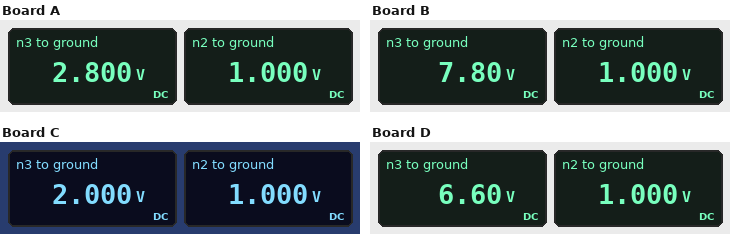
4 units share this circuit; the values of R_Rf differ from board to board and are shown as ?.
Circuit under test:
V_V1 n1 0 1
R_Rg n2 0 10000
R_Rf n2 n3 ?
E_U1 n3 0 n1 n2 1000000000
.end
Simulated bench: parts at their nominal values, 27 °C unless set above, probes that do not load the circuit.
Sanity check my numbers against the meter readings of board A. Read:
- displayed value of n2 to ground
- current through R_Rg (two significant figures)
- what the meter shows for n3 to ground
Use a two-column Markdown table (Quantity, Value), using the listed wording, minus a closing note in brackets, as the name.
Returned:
| Quantity | Value |
|---|---|
| displayed value of n2 to ground | 1.000 V |
| current through R_Rg | 100 µA |
| what the meter shows for n3 to ground | 2.800 V |
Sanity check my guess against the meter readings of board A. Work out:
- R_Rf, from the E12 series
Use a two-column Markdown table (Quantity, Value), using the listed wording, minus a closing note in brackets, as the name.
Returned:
| Quantity | Value |
|---|---|
| R_Rf, from the E12 series | 18 kΩ |
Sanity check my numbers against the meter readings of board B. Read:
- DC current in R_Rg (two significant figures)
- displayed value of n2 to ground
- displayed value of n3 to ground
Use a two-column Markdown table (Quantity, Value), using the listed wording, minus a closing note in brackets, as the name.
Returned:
| Quantity | Value |
|---|---|
| DC current in R_Rg | 100 µA |
| displayed value of n2 to ground | 1.000 V |
| displayed value of n3 to ground | 7.80 V |
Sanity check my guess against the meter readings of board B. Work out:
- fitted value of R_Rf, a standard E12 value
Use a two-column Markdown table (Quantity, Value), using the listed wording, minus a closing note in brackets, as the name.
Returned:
| Quantity | Value |
|---|---|
| fitted value of R_Rf, a standard E12 value | 68 kΩ |
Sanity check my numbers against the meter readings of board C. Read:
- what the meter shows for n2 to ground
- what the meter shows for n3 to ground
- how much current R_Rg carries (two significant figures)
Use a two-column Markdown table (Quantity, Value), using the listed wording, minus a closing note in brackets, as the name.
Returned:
| Quantity | Value |
|---|---|
| what the meter shows for n2 to ground | 1.000 V |
| what the meter shows for n3 to ground | 2.000 V |
| how much current R_Rg carries | 100 µA |
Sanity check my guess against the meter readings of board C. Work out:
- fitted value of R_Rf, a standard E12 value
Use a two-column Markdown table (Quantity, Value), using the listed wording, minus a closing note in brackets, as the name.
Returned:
| Quantity | Value |
|---|---|
| fitted value of R_Rf, a standard E12 value | 10 kΩ |
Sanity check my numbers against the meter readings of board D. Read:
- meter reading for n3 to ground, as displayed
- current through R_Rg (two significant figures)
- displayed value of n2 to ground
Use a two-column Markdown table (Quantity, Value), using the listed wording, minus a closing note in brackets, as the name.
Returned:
| Quantity | Value |
|---|---|
| meter reading for n3 to ground, as displayed | 6.60 V |
| current through R_Rg | 100 µA |
| displayed value of n2 to ground | 1.000 V |
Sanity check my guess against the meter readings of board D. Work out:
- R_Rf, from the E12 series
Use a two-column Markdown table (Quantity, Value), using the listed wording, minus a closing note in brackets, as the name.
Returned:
| Quantity | Value |
|---|---|
| R_Rf, from the E12 series | 56 kΩ |
